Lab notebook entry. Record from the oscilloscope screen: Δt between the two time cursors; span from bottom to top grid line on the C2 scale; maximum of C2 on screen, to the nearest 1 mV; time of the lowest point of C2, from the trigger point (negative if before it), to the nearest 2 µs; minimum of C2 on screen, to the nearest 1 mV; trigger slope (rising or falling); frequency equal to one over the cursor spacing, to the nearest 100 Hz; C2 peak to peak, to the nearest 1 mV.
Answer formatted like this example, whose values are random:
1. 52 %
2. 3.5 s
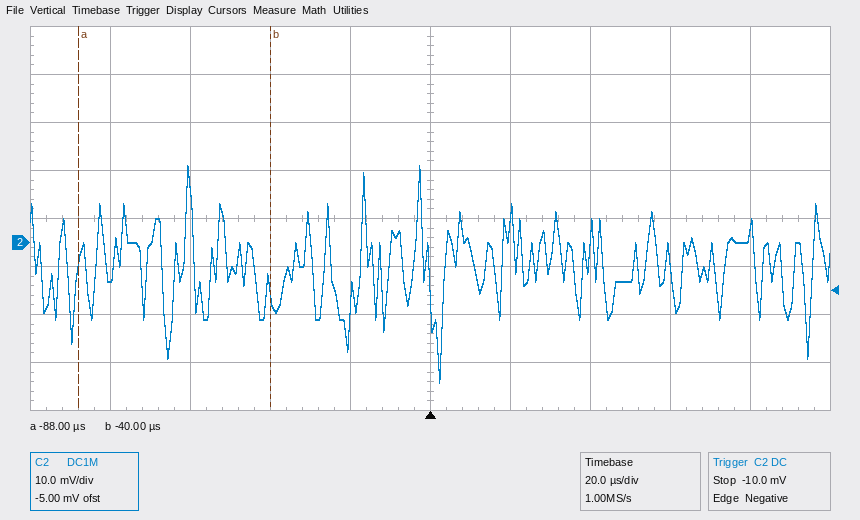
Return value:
1. 48 µs
2. 80 mV
3. 16 mV
4. +2 µs
5. -29 mV
6. falling
7. 20.8 kHz
8. 45 mV
